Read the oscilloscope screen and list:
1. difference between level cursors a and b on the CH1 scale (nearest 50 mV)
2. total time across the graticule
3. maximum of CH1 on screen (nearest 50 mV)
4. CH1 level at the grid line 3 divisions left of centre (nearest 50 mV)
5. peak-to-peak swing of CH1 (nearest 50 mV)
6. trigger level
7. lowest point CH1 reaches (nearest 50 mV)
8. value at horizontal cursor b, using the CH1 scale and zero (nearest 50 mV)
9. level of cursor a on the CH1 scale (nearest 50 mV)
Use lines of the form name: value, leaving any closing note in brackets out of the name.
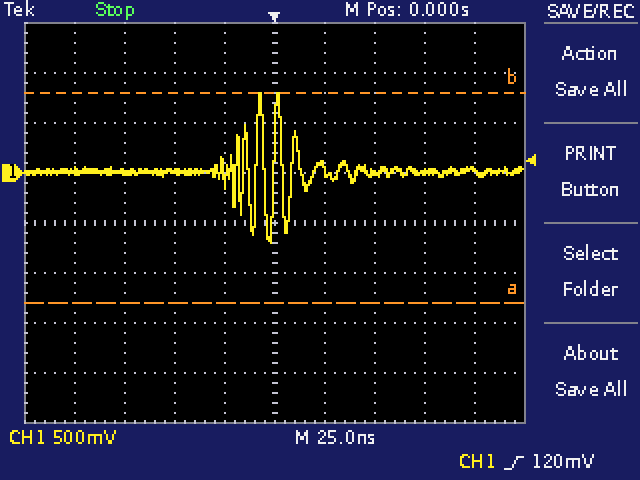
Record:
difference between level cursors a and b on the CH1 scale: 2.10 V
total time across the graticule: 250 ns
maximum of CH1 on screen: 800 mV
CH1 level at the grid line 3 divisions left of centre: 0 mV
peak-to-peak swing of CH1: 1.50 V
trigger level: 120 mV
lowest point CH1 reaches: -700 mV
value at horizontal cursor b, using the CH1 scale and zero: 800 mV
level of cursor a on the CH1 scale: -1.30 V
